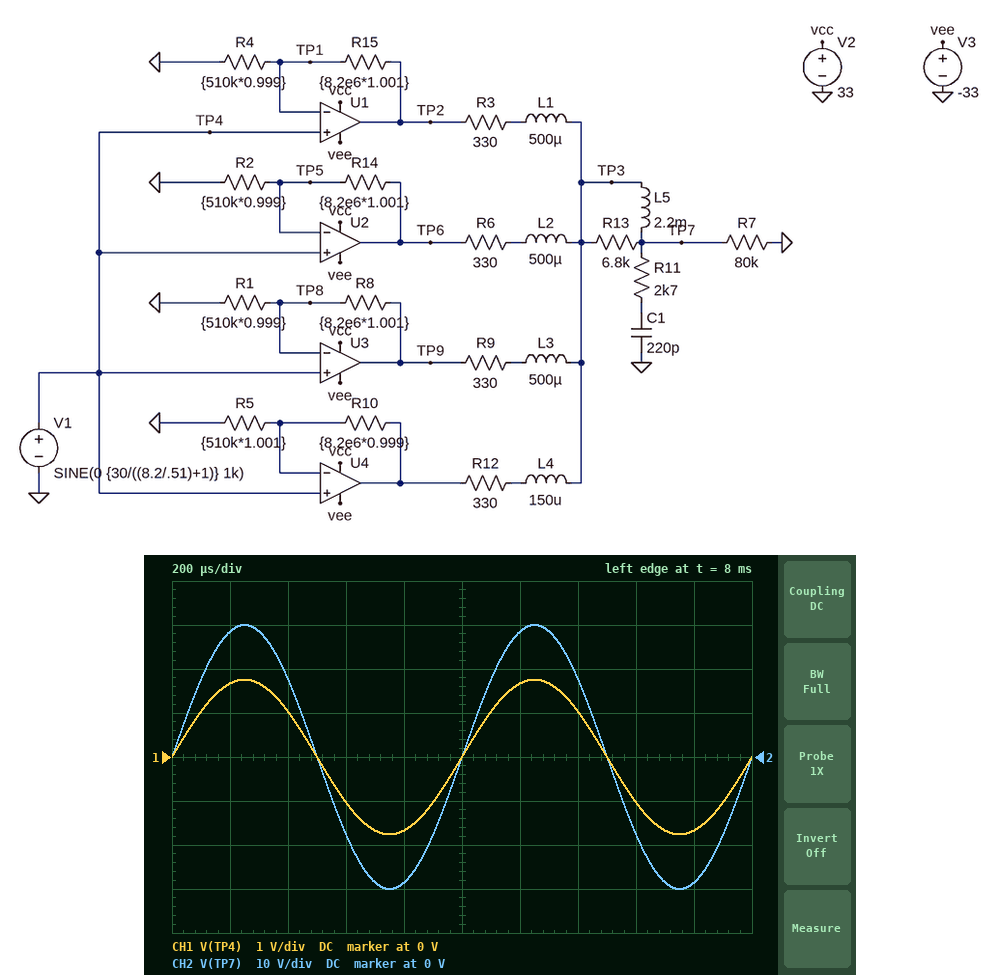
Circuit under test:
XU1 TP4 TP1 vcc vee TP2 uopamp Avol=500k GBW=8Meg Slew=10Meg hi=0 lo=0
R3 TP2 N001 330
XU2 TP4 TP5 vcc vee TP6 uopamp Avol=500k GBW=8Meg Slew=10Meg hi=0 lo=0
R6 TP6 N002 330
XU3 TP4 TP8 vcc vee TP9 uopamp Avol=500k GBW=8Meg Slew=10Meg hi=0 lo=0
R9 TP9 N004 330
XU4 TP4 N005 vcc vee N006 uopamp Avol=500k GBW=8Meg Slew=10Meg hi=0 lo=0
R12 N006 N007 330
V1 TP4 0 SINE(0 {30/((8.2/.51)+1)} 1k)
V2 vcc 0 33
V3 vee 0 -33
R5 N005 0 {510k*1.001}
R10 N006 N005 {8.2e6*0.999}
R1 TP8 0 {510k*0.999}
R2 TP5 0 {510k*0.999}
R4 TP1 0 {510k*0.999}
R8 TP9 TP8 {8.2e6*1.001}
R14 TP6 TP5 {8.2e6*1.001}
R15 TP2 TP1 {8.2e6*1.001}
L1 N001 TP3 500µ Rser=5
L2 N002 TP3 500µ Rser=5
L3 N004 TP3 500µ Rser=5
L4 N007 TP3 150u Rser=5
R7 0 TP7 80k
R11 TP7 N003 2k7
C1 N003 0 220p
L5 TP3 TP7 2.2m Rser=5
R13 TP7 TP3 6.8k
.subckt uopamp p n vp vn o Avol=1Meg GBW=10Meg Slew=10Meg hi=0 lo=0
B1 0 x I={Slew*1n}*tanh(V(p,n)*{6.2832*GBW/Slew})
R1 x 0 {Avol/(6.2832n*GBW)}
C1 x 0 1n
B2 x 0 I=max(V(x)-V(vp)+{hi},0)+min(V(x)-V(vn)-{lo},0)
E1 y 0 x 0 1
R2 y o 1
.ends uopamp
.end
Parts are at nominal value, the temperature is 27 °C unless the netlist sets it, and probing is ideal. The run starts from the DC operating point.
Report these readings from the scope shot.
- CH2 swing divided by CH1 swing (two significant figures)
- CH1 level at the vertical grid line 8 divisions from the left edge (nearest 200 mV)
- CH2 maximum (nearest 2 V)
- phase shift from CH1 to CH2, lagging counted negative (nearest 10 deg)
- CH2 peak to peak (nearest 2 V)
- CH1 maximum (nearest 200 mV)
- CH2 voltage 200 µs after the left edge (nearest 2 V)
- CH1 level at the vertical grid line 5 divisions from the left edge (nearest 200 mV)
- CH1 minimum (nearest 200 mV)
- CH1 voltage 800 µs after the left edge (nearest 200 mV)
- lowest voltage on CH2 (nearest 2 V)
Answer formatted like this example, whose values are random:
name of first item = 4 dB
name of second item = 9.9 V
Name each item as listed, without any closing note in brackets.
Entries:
CH2 swing divided by CH1 swing = 17
CH1 level at the vertical grid line 8 divisions from the left edge = -1.0 V
CH2 maximum = 30 V
phase shift from CH1 to CH2, lagging counted negative = 0 deg
CH2 peak to peak = 60 V
CH1 maximum = 1.8 V
CH2 voltage 200 µs after the left edge = 28 V
CH1 level at the vertical grid line 5 divisions from the left edge = 0 V
CH1 minimum = -1.8 V
CH1 voltage 800 µs after the left edge = -1.6 V
lowest voltage on CH2 = -30 V
